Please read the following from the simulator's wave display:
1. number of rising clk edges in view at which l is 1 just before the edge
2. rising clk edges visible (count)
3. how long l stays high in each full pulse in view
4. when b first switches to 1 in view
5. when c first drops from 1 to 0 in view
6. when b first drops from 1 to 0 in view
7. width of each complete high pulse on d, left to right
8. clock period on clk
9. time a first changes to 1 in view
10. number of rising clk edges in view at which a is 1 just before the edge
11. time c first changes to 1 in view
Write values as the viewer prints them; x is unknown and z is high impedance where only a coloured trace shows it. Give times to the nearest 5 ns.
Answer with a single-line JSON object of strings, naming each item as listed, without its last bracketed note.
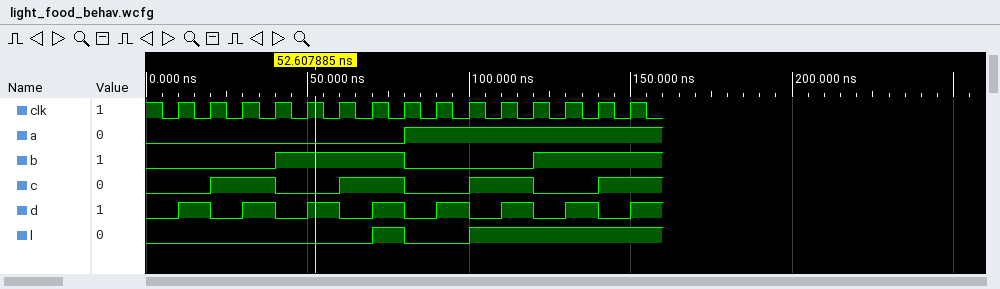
{"number of rising clk edges in view at which l is 1 just before the edge": "6", "rising clk edges visible": "15", "how long l stays high in each full pulse in view": "10 ns", "when b first switches to 1 in view": "40 ns", "when c first drops from 1 to 0 in view": "40 ns", "when b first drops from 1 to 0 in view": "80 ns", "width of each complete high pulse on d, left to right": "10 ns, 10 ns, 10 ns, 10 ns, 10 ns, 10 ns, 10 ns", "clock period on clk": "10 ns", "time a first changes to 1 in view": "80 ns", "number of rising clk edges in view at which a is 1 just before the edge": "7", "time c first changes to 1 in view": "20 ns"}
